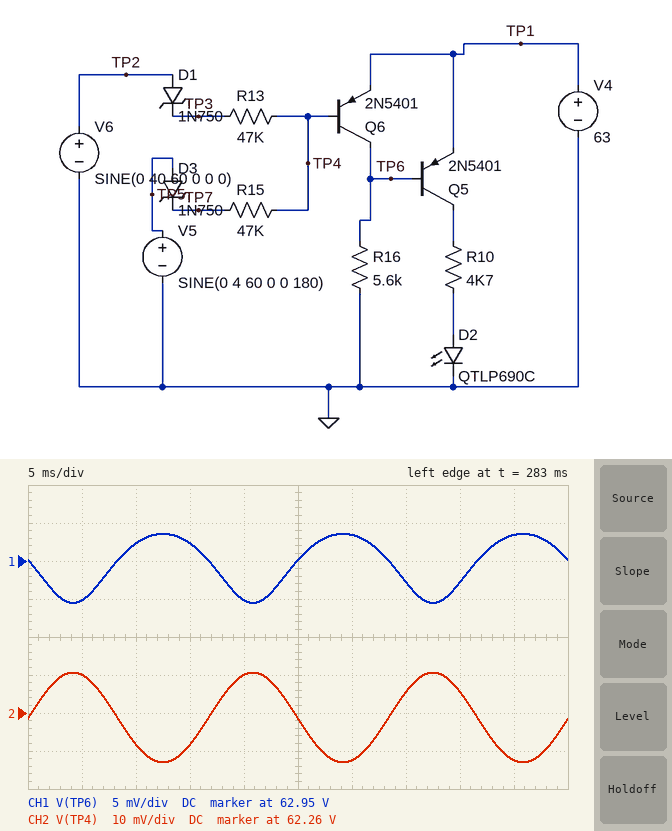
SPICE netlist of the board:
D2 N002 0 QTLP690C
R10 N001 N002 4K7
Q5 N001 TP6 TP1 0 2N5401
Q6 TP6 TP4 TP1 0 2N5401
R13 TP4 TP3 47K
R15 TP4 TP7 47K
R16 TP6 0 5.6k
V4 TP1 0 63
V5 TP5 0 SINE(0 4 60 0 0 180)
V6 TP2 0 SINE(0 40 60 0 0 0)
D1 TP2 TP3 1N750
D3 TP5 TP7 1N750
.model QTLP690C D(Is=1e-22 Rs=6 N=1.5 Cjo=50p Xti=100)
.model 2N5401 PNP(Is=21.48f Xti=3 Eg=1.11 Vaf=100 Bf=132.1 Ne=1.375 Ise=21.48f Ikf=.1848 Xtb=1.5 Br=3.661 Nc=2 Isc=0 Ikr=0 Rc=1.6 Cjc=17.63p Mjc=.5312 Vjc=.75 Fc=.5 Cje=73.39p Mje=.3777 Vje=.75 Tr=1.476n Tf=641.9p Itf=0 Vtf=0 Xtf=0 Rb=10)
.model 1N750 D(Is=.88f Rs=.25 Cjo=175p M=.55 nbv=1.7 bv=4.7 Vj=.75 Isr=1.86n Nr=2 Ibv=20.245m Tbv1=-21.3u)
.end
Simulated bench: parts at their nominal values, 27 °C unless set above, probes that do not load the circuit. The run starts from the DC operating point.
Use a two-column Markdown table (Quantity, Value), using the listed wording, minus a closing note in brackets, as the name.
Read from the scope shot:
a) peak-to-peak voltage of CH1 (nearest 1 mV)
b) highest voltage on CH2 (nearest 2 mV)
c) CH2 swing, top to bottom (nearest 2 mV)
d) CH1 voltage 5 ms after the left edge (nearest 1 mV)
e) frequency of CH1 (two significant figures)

| Quantity | Value |
|---|---|
| peak-to-peak voltage of CH1 | 9 mV |
| highest voltage on CH2 | 62.270 V |
| CH2 swing, top to bottom | 24 mV |
| CH1 voltage 5 ms after the left edge | 62.950 V |
| frequency of CH1 | 60 Hz |
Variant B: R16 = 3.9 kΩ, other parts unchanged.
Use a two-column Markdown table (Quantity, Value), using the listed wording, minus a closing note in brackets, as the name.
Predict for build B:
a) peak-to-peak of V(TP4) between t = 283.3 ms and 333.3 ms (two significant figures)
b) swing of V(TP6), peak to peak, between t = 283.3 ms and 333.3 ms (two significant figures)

| Quantity | Value |
|---|---|
| peak-to-peak of V(TP4) between t = 283.3 ms and 333.3 ms | 22 mV |
| swing of V(TP6), peak to peak, between t = 283.3 ms and 333.3 ms | 11 mV |
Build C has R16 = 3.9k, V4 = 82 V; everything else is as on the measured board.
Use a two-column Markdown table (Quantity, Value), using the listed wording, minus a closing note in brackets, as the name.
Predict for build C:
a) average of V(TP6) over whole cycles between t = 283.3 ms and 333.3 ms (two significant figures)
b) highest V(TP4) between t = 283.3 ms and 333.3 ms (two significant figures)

| Quantity | Value |
|---|---|
| average of V(TP6) over whole cycles between t = 283.3 ms and 333.3 ms | 82 V |
| highest V(TP4) between t = 283.3 ms and 333.3 ms | 81 V |
